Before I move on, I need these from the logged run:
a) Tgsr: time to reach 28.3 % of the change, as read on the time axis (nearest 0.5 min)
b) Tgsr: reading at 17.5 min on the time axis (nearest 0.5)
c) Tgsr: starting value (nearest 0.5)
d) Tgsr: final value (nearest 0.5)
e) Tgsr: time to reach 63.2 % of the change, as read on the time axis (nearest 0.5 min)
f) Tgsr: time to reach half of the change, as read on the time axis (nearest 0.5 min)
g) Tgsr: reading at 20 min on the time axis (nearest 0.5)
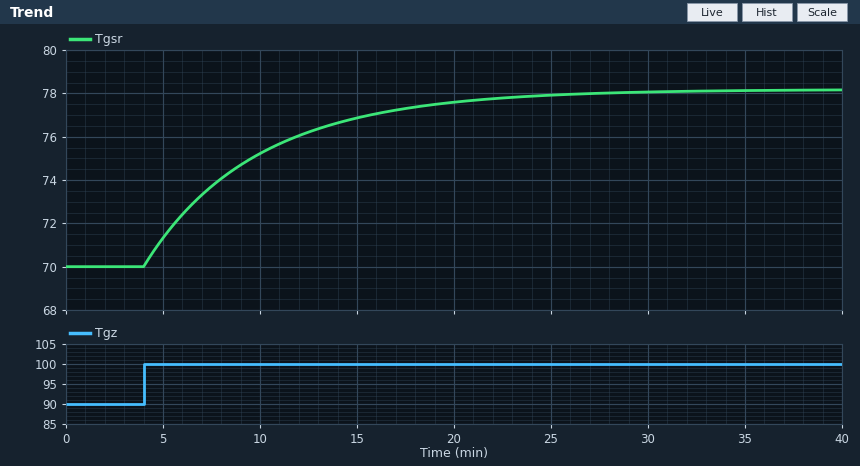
6.0 min
77.5
70.0
78.0
10.0 min
8.0 min
77.5
